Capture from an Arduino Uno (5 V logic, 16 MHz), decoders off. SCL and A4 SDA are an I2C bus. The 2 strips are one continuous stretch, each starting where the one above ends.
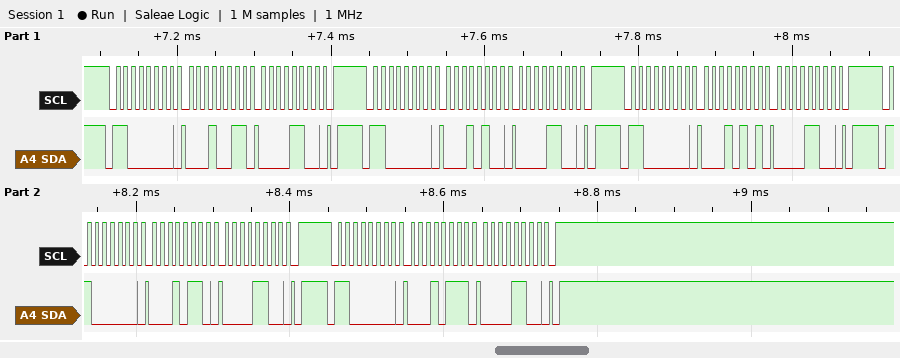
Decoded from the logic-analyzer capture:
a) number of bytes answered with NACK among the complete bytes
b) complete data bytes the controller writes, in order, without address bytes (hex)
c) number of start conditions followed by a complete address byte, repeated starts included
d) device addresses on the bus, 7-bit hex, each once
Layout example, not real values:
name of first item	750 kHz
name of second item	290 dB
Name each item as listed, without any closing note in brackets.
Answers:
number of bytes answered with NACK among the complete bytes	0
complete data bytes the controller writes, in order, without address bytes	13 0C 14 0C 15 0C 16 0C 17 0C
number of start conditions followed by a complete address byte, repeated starts included	5
device addresses on the bus, 7-bit hex, each once	0x60
